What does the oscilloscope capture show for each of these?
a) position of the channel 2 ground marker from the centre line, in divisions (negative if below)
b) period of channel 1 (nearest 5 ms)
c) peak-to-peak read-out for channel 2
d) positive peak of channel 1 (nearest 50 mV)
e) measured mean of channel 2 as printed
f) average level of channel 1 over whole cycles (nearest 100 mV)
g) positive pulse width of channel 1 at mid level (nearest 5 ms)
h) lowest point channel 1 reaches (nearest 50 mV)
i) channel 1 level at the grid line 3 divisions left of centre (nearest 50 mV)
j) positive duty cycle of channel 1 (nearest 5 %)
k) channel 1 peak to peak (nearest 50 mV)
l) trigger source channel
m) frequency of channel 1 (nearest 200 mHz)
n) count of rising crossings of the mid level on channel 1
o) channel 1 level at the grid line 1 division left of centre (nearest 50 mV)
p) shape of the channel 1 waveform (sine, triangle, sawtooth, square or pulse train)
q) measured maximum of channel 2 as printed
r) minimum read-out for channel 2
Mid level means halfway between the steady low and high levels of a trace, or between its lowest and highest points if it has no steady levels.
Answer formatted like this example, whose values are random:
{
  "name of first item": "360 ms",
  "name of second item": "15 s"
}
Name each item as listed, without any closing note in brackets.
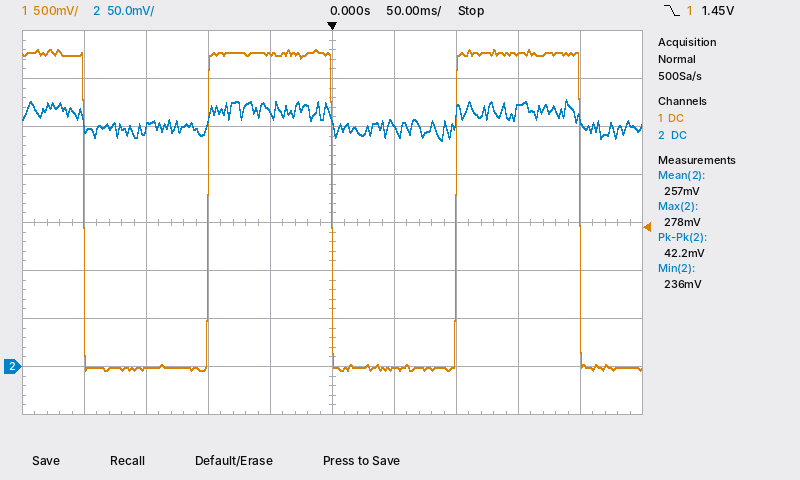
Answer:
{
  "position of the channel 2 ground marker from the centre line, in divisions": "-3.0 div",
  "period of channel 1": "200 ms",
  "peak-to-peak read-out for channel 2": "42.2 mV",
  "positive peak of channel 1": "3.30 V",
  "measured mean of channel 2 as printed": "257 mV",
  "average level of channel 1 over whole cycles": "1.6 V",
  "positive pulse width of channel 1 at mid level": "100 ms",
  "lowest point channel 1 reaches": "-50 mV",
  "channel 1 level at the grid line 3 divisions left of centre": "0 mV",
  "positive duty cycle of channel 1": "50 %",
  "channel 1 peak to peak": "3.35 V",
  "trigger source channel": "channel 1",
  "frequency of channel 1": "5.0 Hz",
  "count of rising crossings of the mid level on channel 1": "2",
  "channel 1 level at the grid line 1 division left of centre": "3.25 V",
  "shape of the channel 1 waveform": "square",
  "measured maximum of channel 2 as printed": "278 mV",
  "minimum read-out for channel 2": "236 mV"
}
